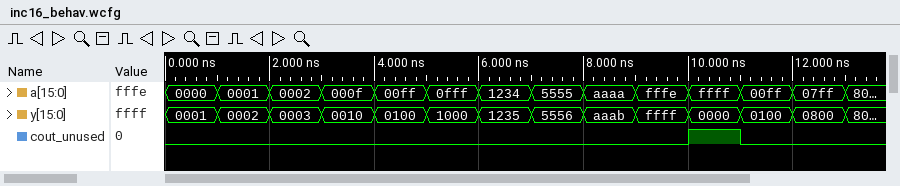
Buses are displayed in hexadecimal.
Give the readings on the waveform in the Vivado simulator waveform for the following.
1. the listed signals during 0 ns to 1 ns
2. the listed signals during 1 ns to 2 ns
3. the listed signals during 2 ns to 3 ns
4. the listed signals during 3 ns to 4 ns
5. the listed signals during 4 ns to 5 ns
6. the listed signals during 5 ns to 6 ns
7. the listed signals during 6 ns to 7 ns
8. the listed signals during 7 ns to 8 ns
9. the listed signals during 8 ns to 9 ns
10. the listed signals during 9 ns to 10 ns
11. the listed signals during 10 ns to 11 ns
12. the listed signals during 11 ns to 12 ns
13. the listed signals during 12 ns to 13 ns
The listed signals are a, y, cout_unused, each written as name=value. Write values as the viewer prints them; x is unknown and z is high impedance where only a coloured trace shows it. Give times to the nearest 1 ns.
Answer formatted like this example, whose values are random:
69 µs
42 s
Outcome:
a=0000, y=0001, cout_unused=0
a=0001, y=0002, cout_unused=0
a=0002, y=0003, cout_unused=0
a=000f, y=0010, cout_unused=0
a=00ff, y=0100, cout_unused=0
a=0fff, y=1000, cout_unused=0
a=1234, y=1235, cout_unused=0
a=5555, y=5556, cout_unused=0
a=aaaa, y=aaab, cout_unused=0
a=fffe, y=ffff, cout_unused=0
a=ffff, y=0000, cout_unused=1
a=00ff, y=0100, cout_unused=0
a=07ff, y=0800, cout_unused=0
